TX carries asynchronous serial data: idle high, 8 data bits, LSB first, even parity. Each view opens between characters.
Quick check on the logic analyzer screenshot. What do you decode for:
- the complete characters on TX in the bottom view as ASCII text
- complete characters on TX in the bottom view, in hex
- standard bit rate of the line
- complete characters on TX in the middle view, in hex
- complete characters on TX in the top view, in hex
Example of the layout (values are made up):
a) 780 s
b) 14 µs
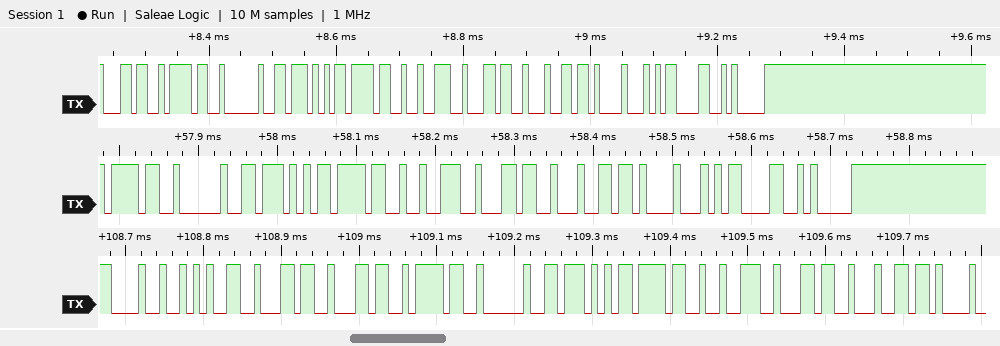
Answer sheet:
a) "Hello World"
b) 48, 65, 6C, 6C, 6F, 20, 57, 6F, 72, 6C, 64
c) 115200 baud
d) 6F, 20, 57, 6F, 72, 6C, 64, 21, 0D, 0A
e) 6C, 6F, 20, 57, 6F, 72, 6C, 64, 21, 0D, 0A
